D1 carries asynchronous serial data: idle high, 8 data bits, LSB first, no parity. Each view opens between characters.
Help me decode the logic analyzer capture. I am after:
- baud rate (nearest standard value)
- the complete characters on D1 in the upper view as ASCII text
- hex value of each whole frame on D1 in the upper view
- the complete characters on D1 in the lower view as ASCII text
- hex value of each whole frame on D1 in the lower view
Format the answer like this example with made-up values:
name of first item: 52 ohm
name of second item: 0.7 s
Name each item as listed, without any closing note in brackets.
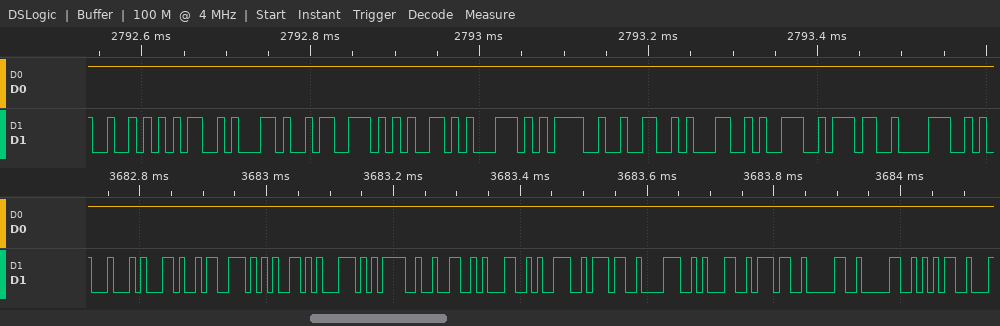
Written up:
baud rate: 115200 baud
the complete characters on D1 in the upper view as ASCII text: "RM,seq=21978"
hex value of each whole frame on D1 in the upper view: 52, 4D, 2C, 73, 65, 71, 3D, 32, 31, 39, 37, 38
the complete characters on D1 in the lower view as ASCII text: "D,seq=2197817005"
hex value of each whole frame on D1 in the lower view: 44, 2C, 73, 65, 71, 3D, 32, 31, 39, 37, 38, 31, 37, 30, 30, 35
